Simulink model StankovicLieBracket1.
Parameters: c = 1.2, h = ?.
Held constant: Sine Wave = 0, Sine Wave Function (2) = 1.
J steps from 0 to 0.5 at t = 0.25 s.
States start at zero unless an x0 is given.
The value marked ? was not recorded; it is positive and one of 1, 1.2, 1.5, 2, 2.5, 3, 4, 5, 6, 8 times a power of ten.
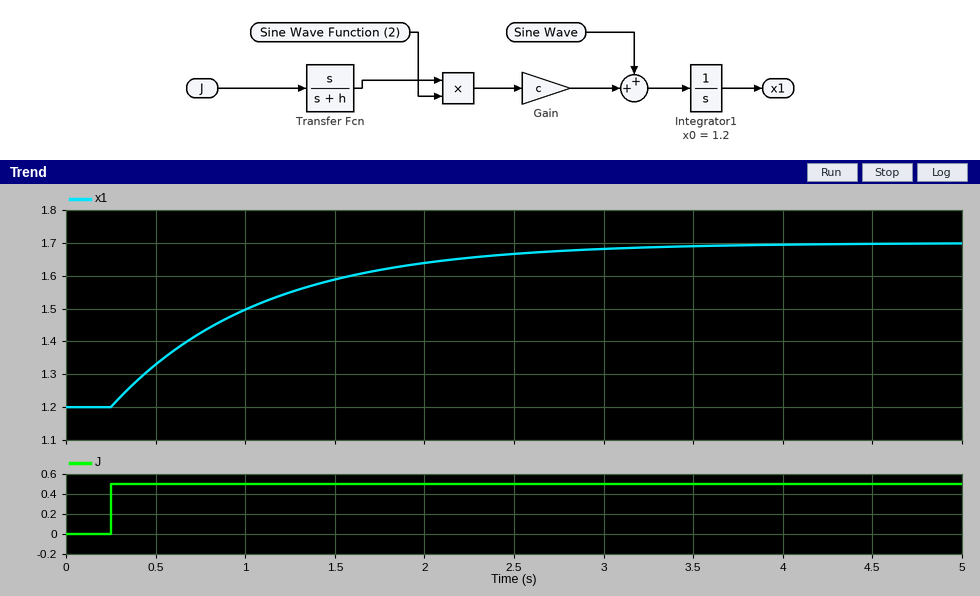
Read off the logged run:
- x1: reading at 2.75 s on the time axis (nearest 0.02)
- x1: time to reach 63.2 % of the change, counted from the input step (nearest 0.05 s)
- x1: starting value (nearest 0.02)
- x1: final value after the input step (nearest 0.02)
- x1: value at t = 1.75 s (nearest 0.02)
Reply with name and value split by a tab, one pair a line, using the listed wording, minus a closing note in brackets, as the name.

x1: reading at 2.75 s on the time axis	1.68
x1: time to reach 63.2 % of the change, counted from the input step	0.85 s
x1: starting value	1.20
x1: final value after the input step	1.70
x1: value at t = 1.75 s	1.62
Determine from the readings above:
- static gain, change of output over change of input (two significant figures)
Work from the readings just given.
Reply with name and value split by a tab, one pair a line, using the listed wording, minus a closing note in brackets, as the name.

static gain, change of output over change of input	1.0
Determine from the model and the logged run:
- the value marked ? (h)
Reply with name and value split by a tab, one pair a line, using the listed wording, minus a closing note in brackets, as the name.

the value marked ?	1.2
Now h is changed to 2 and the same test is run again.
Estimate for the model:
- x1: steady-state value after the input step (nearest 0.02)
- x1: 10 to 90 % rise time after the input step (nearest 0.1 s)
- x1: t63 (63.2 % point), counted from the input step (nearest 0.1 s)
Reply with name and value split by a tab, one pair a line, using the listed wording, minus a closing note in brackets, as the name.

x1: steady-state value after the input step	1.50
x1: 10 to 90 % rise time after the input step	1.1 s
x1: t63 (63.2 % point), counted from the input step	0.5 s
